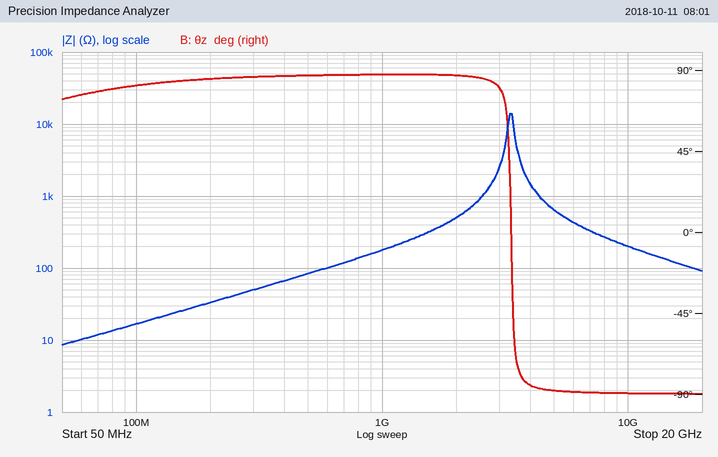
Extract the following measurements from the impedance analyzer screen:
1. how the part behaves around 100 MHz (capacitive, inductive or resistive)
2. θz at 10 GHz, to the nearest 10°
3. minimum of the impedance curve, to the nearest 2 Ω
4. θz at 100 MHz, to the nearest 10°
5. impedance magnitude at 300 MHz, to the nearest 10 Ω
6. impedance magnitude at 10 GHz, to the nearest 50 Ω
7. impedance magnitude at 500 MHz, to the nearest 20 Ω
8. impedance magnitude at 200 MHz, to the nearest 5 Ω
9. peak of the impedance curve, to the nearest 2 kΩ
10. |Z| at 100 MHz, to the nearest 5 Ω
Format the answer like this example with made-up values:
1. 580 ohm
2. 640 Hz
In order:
1. inductive
2. -90°
3. 8 Ω
4. 80°
5. 50 Ω
6. 200 Ω
7. 80 Ω
8. 35 Ω
9. 14 kΩ
10. 15 Ω
